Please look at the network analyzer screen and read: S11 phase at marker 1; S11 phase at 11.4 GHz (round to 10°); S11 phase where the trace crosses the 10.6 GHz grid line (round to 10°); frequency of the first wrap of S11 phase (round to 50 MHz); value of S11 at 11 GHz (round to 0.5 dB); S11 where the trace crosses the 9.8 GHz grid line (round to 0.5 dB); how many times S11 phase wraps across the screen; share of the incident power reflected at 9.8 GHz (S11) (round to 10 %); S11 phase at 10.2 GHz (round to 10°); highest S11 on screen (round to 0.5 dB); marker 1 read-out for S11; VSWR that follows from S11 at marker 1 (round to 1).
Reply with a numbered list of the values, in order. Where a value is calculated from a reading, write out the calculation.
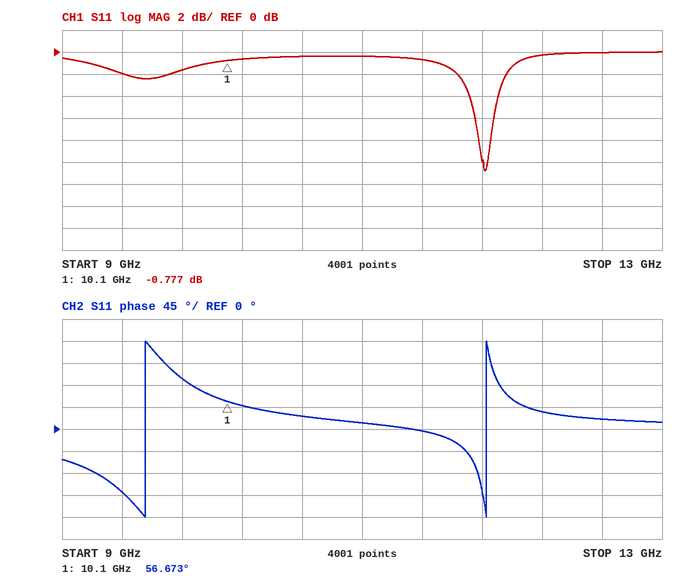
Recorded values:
1. 56.673°
2. 0°
3. 30°
4. 9.55 GHz
5. -0.5 dB
6. -1.5 dB
7. 2
8. 10^(-1.5/10) ≈ 70.8 %, so 70 % to the nearest 10 %
9. 50°
10. 0.0 dB
11. -0.777 dB
12. (1 + 0.9144)/(1 − 0.9144) ≈ 22
